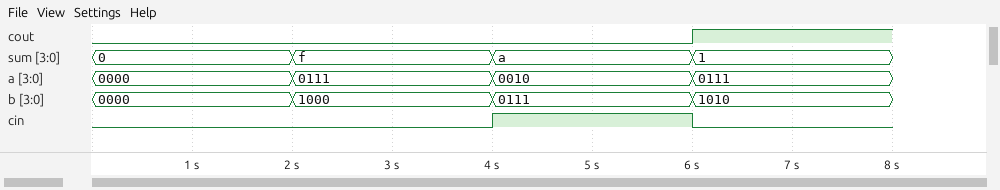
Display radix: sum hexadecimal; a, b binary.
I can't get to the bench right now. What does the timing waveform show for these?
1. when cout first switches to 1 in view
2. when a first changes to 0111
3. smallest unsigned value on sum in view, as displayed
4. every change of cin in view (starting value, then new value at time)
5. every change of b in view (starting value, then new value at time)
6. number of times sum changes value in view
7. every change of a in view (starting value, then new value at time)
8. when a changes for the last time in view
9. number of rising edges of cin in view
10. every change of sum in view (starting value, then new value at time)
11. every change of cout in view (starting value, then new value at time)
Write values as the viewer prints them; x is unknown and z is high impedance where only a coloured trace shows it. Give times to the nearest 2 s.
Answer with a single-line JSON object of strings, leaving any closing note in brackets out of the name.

{"when cout first switches to 1 in view": "6 s", "when a first changes to 0111": "2 s", "smallest unsigned value on sum in view, as displayed": "0", "every change of cin in view": "0, 1 at 4 s, 0 at 6 s", "every change of b in view": "0000, 1000 at 2 s, 0111 at 4 s, 1010 at 6 s", "number of times sum changes value in view": "3", "every change of a in view": "0000, 0111 at 2 s, 0010 at 4 s, 0111 at 6 s", "when a changes for the last time in view": "6 s", "number of rising edges of cin in view": "1", "every change of sum in view": "0, f at 2 s, a at 4 s, 1 at 6 s", "every change of cout in view": "0, 1 at 6 s"}
